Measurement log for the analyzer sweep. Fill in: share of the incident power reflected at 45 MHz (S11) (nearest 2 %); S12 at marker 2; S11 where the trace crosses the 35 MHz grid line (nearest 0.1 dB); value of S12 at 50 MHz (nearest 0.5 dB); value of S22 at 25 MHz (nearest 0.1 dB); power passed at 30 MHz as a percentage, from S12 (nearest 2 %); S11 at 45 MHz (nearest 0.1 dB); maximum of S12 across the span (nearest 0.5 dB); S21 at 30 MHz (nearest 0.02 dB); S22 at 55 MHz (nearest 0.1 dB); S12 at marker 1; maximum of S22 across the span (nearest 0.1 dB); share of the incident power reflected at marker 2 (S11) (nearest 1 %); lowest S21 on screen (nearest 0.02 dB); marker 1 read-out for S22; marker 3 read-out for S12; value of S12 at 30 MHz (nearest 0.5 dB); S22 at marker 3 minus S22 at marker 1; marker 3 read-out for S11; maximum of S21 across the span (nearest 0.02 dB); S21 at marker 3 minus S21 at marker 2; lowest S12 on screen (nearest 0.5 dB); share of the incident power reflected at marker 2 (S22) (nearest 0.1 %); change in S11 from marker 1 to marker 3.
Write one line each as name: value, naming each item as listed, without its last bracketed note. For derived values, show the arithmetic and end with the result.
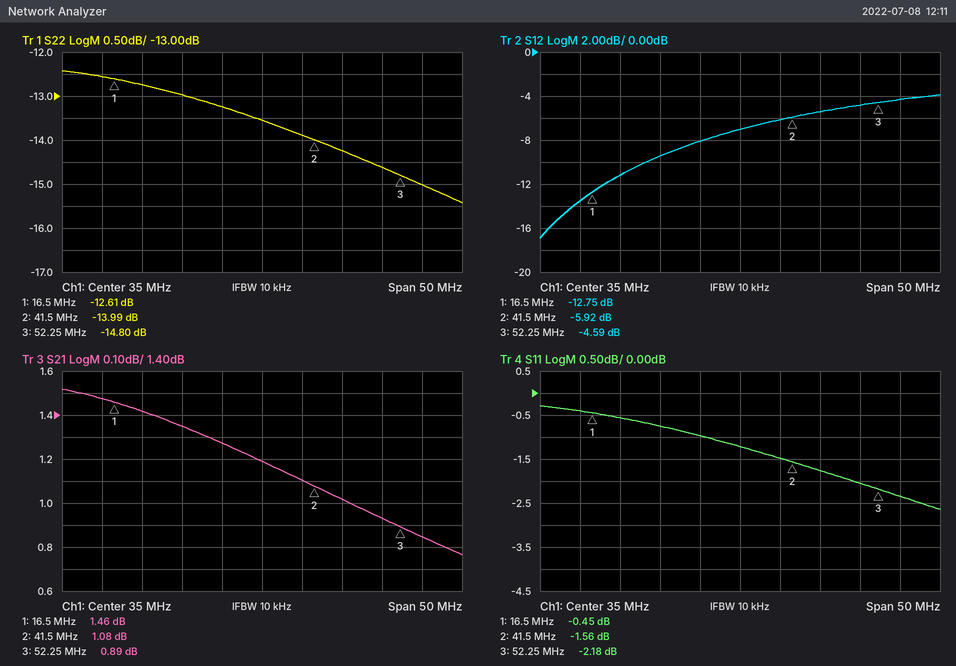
share of the incident power reflected at 45 MHz (S11): 10^(-1.8/10) ≈ 66 %
S12 at marker 2: -5.92 dB
S11 where the trace crosses the 35 MHz grid line: -1.2 dB
value of S12 at 50 MHz: -5.0 dB
value of S22 at 25 MHz: -13.0 dB
power passed at 30 MHz as a percentage, from S12: 10^(-8/10) ≈ 16 %
S11 at 45 MHz: -1.8 dB
maximum of S12 across the span: -4.0 dB
S21 at 30 MHz: 1.28 dB
S22 at 55 MHz: -15.0 dB
S12 at marker 1: -12.75 dB
maximum of S22 across the span: -12.4 dB
share of the incident power reflected at marker 2 (S11): 10^(-1.56/10) ≈ 70 %
lowest S21 on screen: 0.76 dB
marker 1 read-out for S22: -12.61 dB
marker 3 read-out for S12: -4.59 dB
value of S12 at 30 MHz: -8.0 dB
S22 at marker 3 minus S22 at marker 1: -14.8 − (-12.61) = -2.19 dB
marker 3 read-out for S11: -2.18 dB
maximum of S21 across the span: 1.52 dB
S21 at marker 3 minus S21 at marker 2: 0.89 − (1.08) = -0.19 dB
lowest S12 on screen: -17.0 dB
share of the incident power reflected at marker 2 (S22): 10^(-13.99/10) ≈ 4.0 %
change in S11 from marker 1 to marker 3: -2.18 − (-0.45) = -1.73 dB
